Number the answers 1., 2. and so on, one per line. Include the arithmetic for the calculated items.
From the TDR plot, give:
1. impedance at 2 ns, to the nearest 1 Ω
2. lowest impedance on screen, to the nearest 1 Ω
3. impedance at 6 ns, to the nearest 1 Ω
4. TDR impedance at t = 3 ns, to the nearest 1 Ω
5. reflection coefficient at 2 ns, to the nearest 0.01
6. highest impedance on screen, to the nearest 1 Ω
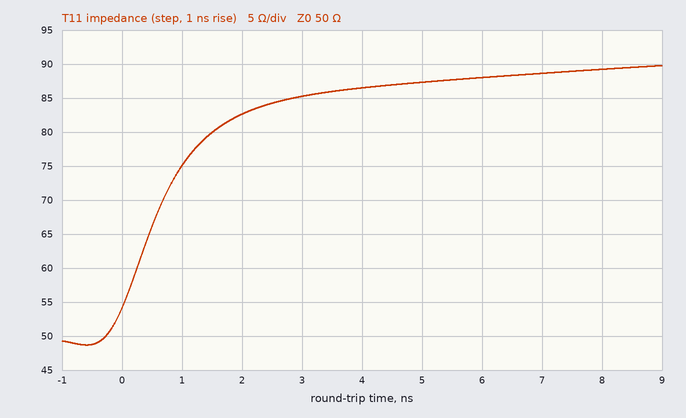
1. 83 Ω
2. 49 Ω
3. 88 Ω
4. 85 Ω
5. (83 − 50)/(83 + 50) ≈ +0.25
6. 90 Ω
